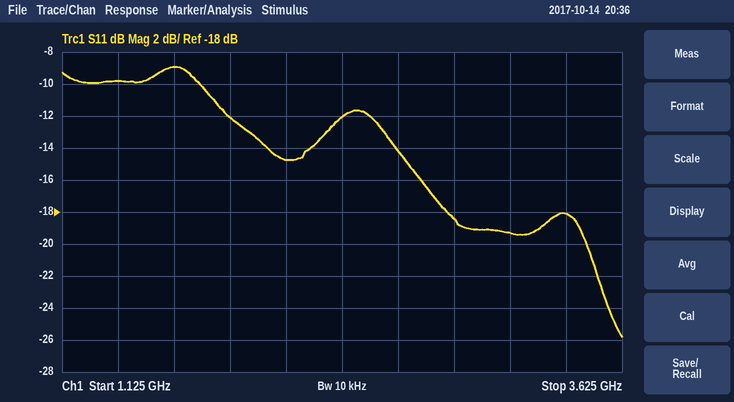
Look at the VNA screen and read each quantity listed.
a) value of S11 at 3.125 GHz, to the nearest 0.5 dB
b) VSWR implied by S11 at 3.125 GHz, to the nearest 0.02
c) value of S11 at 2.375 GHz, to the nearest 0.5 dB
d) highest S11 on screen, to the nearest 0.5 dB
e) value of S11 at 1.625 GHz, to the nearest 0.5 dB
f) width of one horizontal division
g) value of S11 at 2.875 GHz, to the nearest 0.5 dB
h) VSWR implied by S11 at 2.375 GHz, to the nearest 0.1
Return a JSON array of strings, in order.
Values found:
["-19.5 dB", "1.24", "-12.0 dB", "-9.0 dB", "-9.0 dB", "250 MHz", "-18.5 dB", "1.7"]
